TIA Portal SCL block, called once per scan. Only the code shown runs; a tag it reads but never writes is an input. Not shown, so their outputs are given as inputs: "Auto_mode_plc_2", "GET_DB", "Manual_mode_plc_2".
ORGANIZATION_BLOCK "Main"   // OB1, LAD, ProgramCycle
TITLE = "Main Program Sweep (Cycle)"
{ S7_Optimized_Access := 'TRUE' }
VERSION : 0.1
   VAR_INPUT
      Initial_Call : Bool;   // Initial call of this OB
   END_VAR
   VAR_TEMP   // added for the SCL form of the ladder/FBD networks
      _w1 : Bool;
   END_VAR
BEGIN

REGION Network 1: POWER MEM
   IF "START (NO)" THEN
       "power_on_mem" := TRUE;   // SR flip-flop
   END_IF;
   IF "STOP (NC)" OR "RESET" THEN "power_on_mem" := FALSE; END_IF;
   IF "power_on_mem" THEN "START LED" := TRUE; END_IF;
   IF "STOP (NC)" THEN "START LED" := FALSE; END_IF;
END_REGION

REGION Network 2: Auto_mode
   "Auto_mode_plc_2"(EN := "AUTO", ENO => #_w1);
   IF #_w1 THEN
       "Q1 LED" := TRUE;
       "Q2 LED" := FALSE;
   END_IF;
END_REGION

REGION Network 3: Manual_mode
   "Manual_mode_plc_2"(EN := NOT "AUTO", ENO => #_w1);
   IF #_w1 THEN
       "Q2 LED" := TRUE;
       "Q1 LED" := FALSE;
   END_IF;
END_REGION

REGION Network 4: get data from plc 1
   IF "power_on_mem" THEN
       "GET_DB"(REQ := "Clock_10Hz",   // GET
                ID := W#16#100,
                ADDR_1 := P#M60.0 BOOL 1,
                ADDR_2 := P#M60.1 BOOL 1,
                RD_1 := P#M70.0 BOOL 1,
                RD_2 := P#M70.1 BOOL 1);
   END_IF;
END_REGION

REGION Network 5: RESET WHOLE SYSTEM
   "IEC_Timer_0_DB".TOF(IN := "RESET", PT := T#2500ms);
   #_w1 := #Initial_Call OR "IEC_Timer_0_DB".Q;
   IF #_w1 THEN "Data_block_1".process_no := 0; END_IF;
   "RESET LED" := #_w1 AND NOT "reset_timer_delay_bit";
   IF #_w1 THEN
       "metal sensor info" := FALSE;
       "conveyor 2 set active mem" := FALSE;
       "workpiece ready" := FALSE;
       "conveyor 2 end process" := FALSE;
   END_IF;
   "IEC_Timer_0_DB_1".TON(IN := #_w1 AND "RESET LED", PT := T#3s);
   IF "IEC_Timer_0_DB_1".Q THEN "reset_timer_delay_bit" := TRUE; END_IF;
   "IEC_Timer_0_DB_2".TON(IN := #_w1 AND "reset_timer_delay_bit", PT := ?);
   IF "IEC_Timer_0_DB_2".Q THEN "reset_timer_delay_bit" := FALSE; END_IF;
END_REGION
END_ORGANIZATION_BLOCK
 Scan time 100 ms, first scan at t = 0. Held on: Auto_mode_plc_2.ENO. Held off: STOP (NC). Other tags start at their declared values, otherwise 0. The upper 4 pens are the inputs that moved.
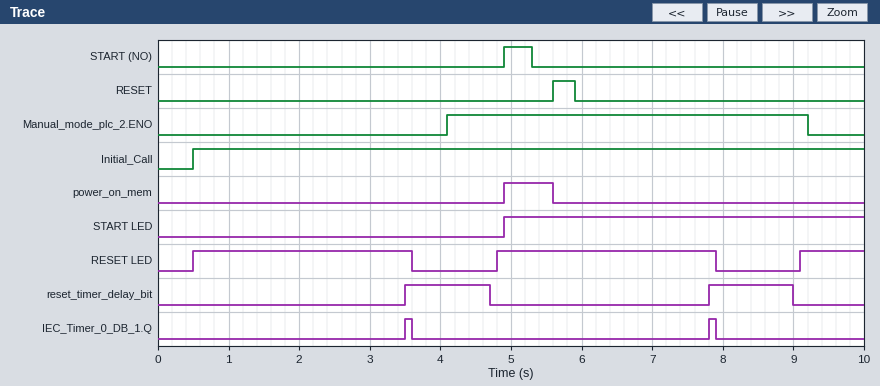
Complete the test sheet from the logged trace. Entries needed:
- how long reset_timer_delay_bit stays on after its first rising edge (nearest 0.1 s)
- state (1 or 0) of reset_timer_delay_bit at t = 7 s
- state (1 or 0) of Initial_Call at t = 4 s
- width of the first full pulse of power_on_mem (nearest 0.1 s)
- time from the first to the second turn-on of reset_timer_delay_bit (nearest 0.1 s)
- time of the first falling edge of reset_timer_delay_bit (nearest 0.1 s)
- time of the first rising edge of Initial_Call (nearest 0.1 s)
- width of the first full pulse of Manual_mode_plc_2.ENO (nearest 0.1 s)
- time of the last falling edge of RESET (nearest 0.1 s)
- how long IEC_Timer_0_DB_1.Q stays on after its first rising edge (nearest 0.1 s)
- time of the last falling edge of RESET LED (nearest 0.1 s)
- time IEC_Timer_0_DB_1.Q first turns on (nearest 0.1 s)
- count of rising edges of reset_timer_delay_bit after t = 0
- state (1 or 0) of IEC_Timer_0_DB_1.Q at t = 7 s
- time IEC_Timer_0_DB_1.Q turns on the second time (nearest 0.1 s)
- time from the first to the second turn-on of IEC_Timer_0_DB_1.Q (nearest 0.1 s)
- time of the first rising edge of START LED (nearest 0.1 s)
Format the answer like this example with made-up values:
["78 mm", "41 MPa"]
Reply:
["1.2 s", "0", "1", "0.7 s", "4.3 s", "4.7 s", "0.5 s", "5.1 s", "5.9 s", "0.1 s", "7.9 s", "3.5 s", "2", "0", "7.8 s", "4.3 s", "4.9 s"]
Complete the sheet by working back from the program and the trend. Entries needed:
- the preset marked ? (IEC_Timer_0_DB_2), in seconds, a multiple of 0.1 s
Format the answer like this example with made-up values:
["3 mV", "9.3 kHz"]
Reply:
["1.2 s"]
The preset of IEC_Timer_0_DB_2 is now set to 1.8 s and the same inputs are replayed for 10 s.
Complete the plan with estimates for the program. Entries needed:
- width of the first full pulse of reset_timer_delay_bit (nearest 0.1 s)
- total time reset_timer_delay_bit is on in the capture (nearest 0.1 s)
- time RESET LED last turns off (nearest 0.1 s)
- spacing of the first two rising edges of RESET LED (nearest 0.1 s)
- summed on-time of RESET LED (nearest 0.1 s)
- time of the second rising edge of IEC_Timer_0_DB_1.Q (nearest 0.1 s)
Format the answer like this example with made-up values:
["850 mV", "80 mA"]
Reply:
["1.8 s", "3.4 s", "8.5 s", "4.9 s", "6.2 s", "8.4 s"]
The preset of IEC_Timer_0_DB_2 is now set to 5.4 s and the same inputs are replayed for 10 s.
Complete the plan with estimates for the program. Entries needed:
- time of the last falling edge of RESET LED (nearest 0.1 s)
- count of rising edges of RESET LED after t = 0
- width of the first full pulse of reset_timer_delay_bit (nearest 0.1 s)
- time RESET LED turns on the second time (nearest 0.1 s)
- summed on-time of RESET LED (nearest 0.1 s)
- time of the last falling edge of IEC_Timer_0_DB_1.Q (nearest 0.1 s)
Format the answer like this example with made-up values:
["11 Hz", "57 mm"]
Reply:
["3.6 s", "2", "5.4 s", "9.0 s", "4.1 s", "3.6 s"]
